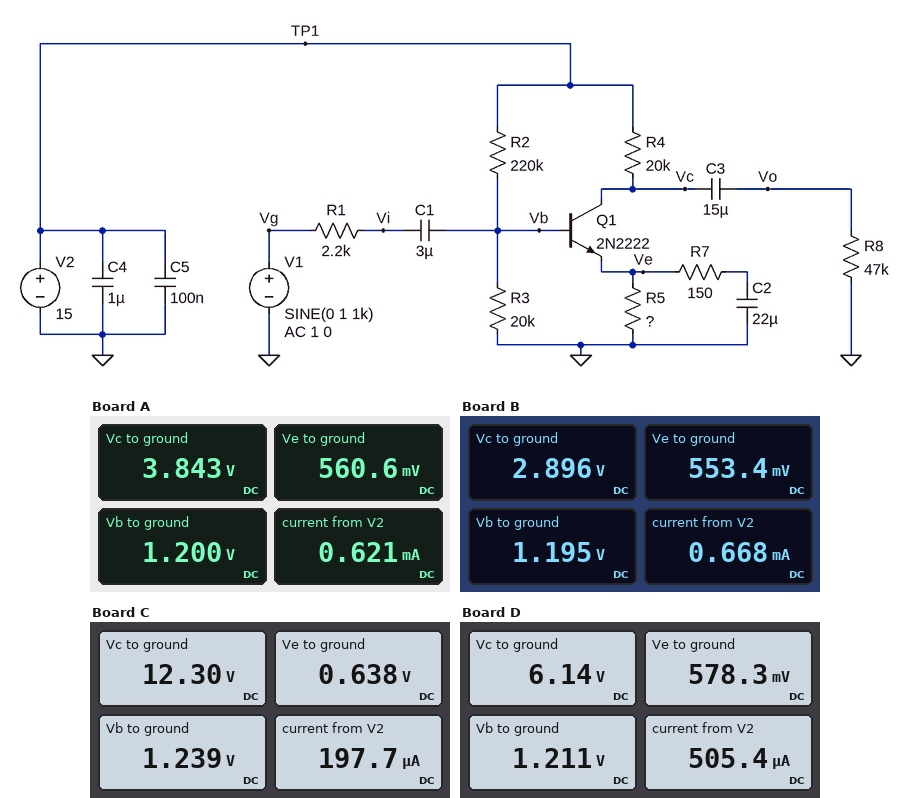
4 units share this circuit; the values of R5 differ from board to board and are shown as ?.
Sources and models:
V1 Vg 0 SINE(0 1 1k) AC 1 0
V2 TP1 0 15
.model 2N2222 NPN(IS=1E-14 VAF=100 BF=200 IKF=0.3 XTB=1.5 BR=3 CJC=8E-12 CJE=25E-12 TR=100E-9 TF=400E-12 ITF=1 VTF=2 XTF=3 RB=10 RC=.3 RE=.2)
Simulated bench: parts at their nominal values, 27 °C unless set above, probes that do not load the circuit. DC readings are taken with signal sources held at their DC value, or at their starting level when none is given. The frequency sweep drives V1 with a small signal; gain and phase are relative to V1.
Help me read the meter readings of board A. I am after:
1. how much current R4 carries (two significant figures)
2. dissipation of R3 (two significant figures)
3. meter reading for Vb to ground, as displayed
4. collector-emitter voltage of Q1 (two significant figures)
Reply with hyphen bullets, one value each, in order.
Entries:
- 560 µA
- 72 µW
- 1.200 V
- 3.3 V
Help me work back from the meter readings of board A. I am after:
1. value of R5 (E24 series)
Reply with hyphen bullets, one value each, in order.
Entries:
- 1 kΩ
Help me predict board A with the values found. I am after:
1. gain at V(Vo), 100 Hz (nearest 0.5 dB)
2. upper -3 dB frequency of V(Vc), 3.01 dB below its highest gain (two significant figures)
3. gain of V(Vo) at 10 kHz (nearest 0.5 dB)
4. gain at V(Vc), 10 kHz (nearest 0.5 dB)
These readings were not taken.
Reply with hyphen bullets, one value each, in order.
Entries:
- 36.0 dB
- 200 kHz
- 36.5 dB
- 36.5 dB
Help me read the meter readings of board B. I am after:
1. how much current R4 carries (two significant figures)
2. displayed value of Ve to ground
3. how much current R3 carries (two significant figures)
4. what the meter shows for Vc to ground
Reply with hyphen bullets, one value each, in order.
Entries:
- 610 µA
- 553.4 mV
- 60 µA
- 2.896 V
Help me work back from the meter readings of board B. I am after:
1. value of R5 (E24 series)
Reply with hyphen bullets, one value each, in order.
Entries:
- 910 Ω
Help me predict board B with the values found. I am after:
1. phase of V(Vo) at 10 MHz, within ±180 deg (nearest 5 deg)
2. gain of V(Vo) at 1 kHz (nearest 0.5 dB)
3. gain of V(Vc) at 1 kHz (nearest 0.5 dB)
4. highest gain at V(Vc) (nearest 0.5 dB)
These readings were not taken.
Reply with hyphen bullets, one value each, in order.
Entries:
- 80 deg
- 36.5 dB
- 36.5 dB
- 36.5 dB
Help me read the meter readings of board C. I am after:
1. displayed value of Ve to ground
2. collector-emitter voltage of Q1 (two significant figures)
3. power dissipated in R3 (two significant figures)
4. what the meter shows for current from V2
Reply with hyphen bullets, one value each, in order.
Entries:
- 0.638 V
- 12 V
- 77 µW
- 197.7 µA
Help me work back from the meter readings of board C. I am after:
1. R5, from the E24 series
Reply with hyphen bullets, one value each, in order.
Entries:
- 4.7 kΩ
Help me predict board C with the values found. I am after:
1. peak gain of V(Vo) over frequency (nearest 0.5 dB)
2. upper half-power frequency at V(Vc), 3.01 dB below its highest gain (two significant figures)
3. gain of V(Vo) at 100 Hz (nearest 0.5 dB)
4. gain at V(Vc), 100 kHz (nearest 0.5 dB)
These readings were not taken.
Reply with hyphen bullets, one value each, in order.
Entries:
- 31.0 dB
- 460 kHz
- 31.0 dB
- 31.0 dB
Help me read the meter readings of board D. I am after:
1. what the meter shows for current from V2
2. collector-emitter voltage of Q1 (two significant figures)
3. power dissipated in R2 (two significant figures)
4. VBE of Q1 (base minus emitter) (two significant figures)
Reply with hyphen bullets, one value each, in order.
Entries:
- 505.4 µA
- 5.6 V
- 860 µW
- 630 mV
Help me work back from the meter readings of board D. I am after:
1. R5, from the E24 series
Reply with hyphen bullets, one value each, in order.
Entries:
- 1.3 kΩ
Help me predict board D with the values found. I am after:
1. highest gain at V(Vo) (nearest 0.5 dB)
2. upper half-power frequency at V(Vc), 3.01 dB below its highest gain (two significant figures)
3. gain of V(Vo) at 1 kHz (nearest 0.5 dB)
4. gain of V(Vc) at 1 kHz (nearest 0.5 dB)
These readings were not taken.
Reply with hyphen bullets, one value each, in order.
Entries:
- 35.5 dB
- 250 kHz
- 35.5 dB
- 35.5 dB
